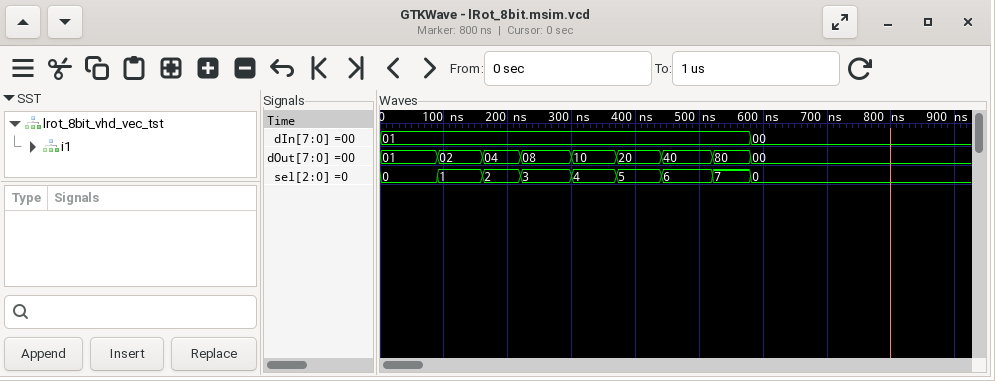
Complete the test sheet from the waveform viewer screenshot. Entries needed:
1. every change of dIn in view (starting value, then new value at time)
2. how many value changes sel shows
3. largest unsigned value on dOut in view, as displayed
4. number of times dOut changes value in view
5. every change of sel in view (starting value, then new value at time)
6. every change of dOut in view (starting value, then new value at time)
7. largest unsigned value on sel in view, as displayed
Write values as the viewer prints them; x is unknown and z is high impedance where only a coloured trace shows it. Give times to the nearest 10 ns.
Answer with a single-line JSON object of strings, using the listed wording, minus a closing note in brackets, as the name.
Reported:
{"every change of dIn in view": "01, 00 at 580 ns", "how many value changes sel shows": "8", "largest unsigned value on dOut in view, as displayed": "80", "number of times dOut changes value in view": "8", "every change of sel in view": "0, 1 at 90 ns, 2 at 160 ns, 3 at 220 ns, 4 at 300 ns, 5 at 370 ns, 6 at 440 ns, 7 at 520 ns, 0 at 580 ns", "every change of dOut in view": "01, 02 at 90 ns, 04 at 160 ns, 08 at 220 ns, 10 at 300 ns, 20 at 370 ns, 40 at 440 ns, 80 at 520 ns, 00 at 580 ns", "largest unsigned value on sel in view, as displayed": "7"}
